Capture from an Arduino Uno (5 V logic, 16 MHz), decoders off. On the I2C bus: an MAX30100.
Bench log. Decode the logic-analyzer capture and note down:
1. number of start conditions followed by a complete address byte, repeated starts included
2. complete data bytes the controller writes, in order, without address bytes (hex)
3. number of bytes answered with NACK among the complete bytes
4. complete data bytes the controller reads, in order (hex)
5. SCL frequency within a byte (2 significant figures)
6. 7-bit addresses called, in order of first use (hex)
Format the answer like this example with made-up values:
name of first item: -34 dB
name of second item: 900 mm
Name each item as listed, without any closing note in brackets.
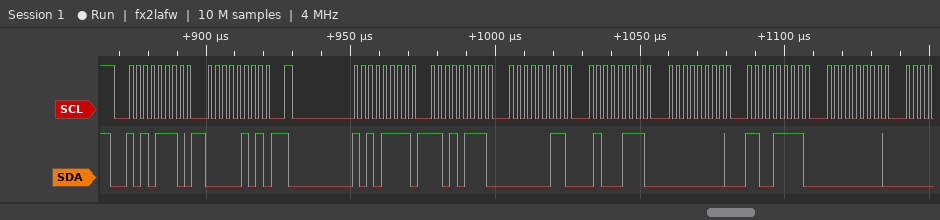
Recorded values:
number of start conditions followed by a complete address byte, repeated starts included: 2
complete data bytes the controller writes, in order, without address bytes: 05
number of bytes answered with NACK among the complete bytes: 0
complete data bytes the controller reads, in order: D7 03 47 00 CF 00
SCL frequency within a byte: 400 kHz
7-bit addresses called, in order of first use: 0x57
